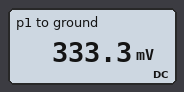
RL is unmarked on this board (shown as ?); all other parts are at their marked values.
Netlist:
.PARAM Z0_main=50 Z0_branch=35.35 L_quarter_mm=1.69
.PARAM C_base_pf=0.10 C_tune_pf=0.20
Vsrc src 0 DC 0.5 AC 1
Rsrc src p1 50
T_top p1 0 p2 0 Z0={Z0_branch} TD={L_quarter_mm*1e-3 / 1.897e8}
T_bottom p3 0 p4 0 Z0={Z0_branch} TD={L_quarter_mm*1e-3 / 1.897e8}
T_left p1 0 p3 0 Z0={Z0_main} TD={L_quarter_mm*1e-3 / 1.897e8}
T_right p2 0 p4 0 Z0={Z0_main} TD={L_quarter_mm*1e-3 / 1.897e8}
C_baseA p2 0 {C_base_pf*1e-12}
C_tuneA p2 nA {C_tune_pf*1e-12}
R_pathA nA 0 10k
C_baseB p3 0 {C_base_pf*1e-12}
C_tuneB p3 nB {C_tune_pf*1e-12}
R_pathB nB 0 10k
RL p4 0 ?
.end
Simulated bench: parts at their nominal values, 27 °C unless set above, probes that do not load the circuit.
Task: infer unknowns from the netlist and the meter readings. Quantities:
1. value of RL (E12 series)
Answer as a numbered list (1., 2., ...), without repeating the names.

1. 100 Ω
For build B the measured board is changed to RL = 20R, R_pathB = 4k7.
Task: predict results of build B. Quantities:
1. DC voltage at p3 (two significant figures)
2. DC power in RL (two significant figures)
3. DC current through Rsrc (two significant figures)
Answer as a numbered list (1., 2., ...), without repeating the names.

1. 140 mV
2. 1.0 mW
3. 7.1 mA
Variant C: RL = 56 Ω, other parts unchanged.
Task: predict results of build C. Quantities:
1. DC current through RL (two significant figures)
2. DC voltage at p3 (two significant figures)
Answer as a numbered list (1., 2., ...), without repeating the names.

1. 4.7 mA
2. 260 mV
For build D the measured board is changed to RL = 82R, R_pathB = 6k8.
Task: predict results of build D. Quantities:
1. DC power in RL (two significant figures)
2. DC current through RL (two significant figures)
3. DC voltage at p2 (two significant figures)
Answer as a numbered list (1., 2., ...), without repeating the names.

1. 1.2 mW
2. 3.8 mA
3. 310 mV
